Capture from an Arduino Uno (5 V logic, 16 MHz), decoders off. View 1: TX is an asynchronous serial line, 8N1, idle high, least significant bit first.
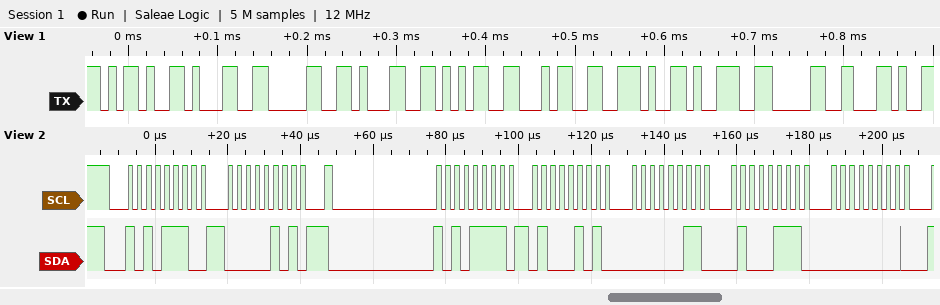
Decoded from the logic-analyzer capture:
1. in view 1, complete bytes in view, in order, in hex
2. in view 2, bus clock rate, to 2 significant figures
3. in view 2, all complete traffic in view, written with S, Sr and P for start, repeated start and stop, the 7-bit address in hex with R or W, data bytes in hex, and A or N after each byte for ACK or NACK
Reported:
2D 31 30 31 35 34 2E 39 30 2C
400 kHz
S 57W A 05 A Sr 57R A 45 A 03 A 47 A 00 A
